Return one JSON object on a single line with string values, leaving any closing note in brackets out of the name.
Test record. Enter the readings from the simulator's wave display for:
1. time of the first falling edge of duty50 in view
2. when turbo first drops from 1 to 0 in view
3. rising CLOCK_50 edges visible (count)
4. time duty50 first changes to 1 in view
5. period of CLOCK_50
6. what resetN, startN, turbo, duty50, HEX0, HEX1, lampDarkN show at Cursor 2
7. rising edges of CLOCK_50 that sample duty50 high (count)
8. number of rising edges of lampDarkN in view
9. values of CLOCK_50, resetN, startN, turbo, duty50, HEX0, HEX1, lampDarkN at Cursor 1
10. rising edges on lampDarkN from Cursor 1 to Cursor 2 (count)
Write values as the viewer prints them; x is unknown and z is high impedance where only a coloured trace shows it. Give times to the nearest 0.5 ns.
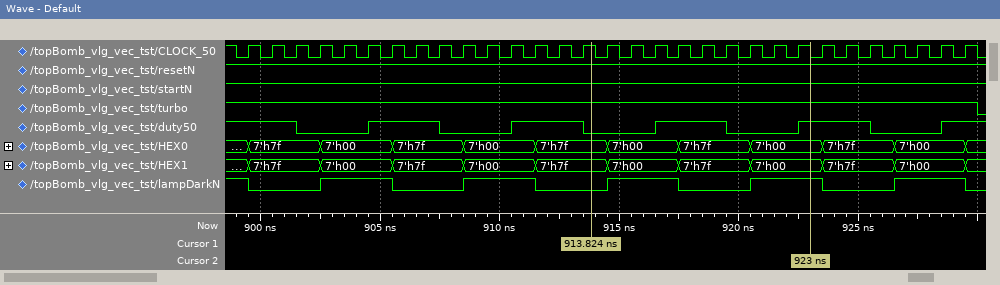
{"time of the first falling edge of duty50 in view": "901.5 ns", "when turbo first drops from 1 to 0 in view": "930 ns", "rising CLOCK_50 edges visible": "31", "time duty50 first changes to 1 in view": "904.5 ns", "period of CLOCK_50": "1 ns", "what resetN, startN, turbo, duty50, HEX0, HEX1, lampDarkN show at Cursor 2": "resetN=1, startN=1, turbo=1, duty50=1, HEX0=7'h00, HEX1=7'h00, lampDarkN=1", "rising edges of CLOCK_50 that sample duty50 high": "16", "number of rising edges of lampDarkN in view": "5", "values of CLOCK_50, resetN, startN, turbo, duty50, HEX0, HEX1, lampDarkN at Cursor 1": "CLOCK_50=1, resetN=1, startN=1, turbo=1, duty50=0, HEX0=7'h7f, HEX1=7'h7f, lampDarkN=0", "rising edges on lampDarkN from Cursor 1 to Cursor 2": "2"}
